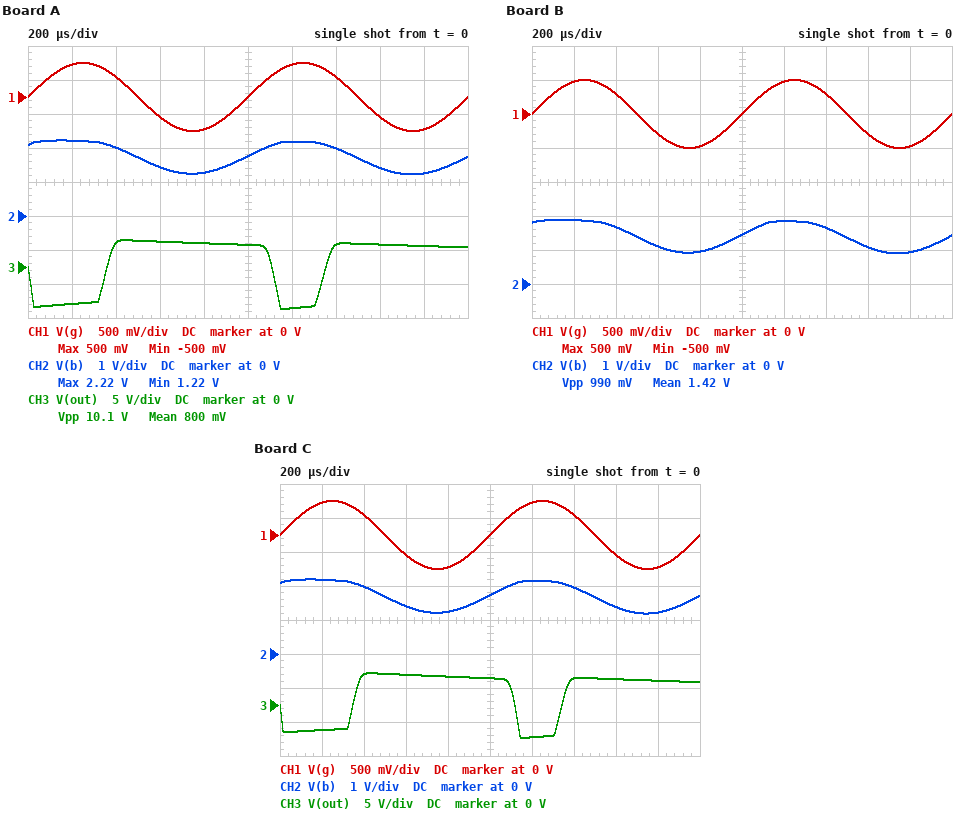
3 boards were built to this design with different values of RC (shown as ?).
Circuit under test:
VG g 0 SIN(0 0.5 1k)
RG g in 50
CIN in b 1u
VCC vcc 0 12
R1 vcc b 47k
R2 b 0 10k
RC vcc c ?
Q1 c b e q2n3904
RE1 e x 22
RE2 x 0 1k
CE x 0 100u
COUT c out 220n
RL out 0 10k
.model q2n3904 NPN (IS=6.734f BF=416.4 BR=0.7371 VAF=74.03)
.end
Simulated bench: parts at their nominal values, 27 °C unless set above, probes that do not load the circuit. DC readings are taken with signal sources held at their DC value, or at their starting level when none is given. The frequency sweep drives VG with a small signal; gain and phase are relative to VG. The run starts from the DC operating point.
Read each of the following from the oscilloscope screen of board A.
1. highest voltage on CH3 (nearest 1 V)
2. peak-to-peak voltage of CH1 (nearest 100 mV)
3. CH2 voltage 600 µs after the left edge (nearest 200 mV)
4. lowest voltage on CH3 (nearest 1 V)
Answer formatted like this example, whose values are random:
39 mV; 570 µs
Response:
4 V; 1.0 V; 1.4 V; -6 V
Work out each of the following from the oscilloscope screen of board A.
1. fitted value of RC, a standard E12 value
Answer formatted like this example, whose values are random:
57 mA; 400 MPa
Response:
3.3 kΩ
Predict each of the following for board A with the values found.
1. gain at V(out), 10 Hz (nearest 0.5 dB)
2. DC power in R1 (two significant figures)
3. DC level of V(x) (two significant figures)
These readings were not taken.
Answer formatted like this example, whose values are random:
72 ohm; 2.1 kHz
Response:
1.0 dB; 2.1 mW; 1.4 V
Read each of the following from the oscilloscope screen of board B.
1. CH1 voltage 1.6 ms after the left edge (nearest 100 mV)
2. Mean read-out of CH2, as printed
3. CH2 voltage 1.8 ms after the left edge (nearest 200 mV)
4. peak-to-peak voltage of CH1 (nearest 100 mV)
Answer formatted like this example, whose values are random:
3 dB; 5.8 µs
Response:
-300 mV; 1.42 V; 1.0 V; 1.0 V
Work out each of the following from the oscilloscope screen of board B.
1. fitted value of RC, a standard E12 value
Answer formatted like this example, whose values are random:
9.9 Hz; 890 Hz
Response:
10 kΩ
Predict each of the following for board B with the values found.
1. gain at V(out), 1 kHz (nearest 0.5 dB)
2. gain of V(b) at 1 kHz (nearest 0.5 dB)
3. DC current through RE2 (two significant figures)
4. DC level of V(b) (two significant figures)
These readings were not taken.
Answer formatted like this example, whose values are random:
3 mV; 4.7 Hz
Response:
11.0 dB; -9.5 dB; 1.1 mA; 1.8 V
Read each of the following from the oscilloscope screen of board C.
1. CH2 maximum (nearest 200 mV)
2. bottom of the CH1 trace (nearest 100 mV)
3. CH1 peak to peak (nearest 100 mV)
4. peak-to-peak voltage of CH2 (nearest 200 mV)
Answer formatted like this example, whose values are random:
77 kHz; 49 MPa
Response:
2.2 V; -500 mV; 1.0 V; 1.0 V
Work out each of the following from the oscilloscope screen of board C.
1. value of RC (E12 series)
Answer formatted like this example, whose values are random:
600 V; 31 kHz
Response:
4.7 kΩ
